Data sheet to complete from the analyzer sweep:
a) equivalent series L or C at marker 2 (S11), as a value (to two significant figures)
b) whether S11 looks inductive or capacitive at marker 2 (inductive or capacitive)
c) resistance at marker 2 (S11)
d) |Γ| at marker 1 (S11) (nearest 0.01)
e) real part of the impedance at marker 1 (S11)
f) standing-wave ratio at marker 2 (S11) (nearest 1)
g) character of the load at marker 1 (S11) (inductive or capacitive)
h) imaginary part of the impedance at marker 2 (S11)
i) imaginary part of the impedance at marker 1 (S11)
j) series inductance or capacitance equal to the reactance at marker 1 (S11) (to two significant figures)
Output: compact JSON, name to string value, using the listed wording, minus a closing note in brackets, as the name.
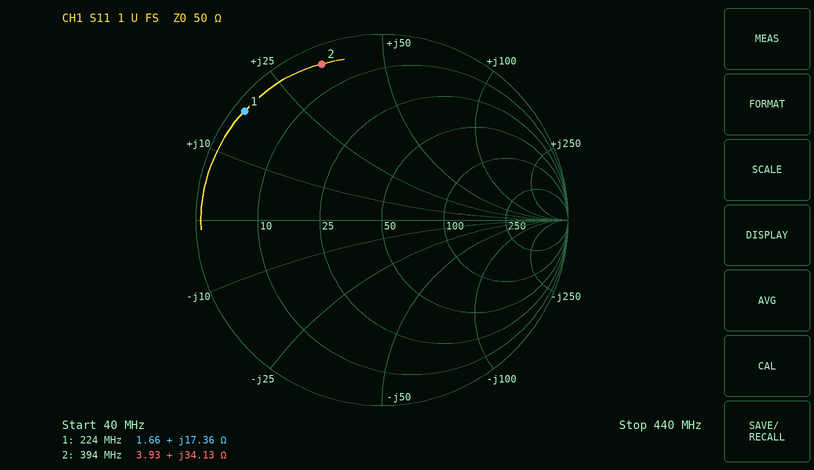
{"equivalent series L or C at marker 2 (S11), as a value": "14 nH", "whether S11 looks inductive or capacitive at marker 2": "inductive", "resistance at marker 2": "3.93 Ω", "|Γ| at marker 1 (S11)": "0.94", "real part of the impedance at marker 1": "1.66 Ω", "standing-wave ratio at marker 2 (S11)": "19", "character of the load at marker 1 (S11)": "inductive", "imaginary part of the impedance at marker 2": "+34.13 Ω", "imaginary part of the impedance at marker 1": "+17.36 Ω", "series inductance or capacitance equal to the reactance at marker 1 (S11)": "12 nH"}
